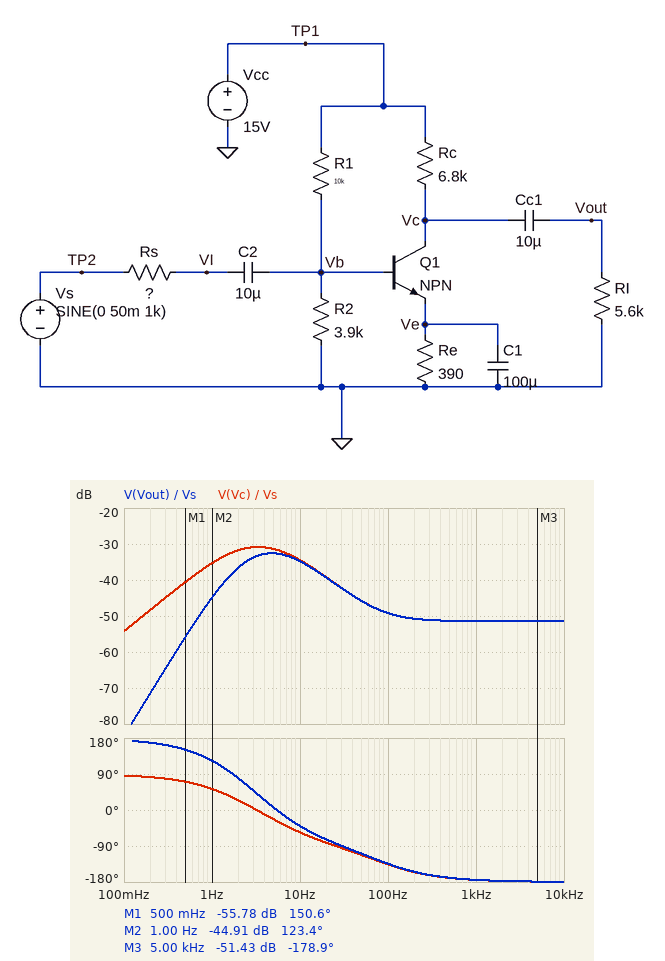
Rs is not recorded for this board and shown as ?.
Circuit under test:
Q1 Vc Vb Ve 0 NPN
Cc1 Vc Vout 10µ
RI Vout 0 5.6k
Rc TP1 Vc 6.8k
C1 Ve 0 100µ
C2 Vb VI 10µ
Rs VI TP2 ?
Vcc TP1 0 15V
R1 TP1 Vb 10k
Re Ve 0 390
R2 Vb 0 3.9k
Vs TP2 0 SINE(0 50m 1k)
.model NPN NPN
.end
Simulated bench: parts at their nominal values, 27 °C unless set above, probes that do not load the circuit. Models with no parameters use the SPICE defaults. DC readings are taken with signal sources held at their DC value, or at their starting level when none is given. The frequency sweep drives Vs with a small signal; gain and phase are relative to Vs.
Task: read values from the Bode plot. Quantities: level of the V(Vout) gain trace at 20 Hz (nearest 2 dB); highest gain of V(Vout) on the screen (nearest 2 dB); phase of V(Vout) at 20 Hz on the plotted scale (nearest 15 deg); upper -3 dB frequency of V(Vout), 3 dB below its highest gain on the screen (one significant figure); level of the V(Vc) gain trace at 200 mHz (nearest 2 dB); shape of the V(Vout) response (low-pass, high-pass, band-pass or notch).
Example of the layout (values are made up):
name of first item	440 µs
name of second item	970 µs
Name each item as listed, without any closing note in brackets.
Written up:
level of the V(Vout) gain trace at 20 Hz	-40 dB
highest gain of V(Vout) on the screen	-32 dB
phase of V(Vout) at 20 Hz on the plotted scale	-75 deg
upper -3 dB frequency of V(Vout), 3 dB below its highest gain on the screen	10 Hz
level of the V(Vc) gain trace at 200 mHz	-48 dB
shape of the V(Vout) response	band-pass
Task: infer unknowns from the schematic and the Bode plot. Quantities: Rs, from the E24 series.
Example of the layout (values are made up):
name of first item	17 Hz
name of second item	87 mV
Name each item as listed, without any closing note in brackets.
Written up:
Rs, from the E24 series	6.8 kΩ
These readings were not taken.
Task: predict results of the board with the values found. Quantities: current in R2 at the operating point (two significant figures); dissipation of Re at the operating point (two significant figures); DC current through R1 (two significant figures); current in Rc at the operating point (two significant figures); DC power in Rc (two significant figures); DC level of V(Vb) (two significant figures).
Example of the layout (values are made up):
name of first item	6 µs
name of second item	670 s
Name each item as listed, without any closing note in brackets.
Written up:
current in R2 at the operating point	490 µA
dissipation of Re at the operating point	3.2 mW
DC current through R1	1.3 mA
current in Rc at the operating point	2.0 mA
DC power in Rc	28 mW
DC level of V(Vb)	1.9 V
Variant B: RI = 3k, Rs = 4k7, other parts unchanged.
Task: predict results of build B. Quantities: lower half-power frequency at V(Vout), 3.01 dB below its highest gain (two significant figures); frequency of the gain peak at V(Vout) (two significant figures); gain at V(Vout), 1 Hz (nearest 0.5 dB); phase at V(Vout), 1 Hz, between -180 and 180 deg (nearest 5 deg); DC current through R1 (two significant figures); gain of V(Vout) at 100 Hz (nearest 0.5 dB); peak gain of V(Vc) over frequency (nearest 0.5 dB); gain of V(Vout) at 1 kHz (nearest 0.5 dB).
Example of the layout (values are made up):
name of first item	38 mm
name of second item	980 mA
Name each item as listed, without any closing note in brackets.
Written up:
lower half-power frequency at V(Vout), 3.01 dB below its highest gain	3.1 Hz
frequency of the gain peak at V(Vout)	6.6 Hz
gain at V(Vout), 1 Hz	-49.5 dB
phase at V(Vout), 1 Hz, between -180 and 180 deg	140 deg
DC current through R1	1.3 mA
gain of V(Vout) at 100 Hz	-46.0 dB
peak gain of V(Vc) over frequency	-29.0 dB
gain of V(Vout) at 1 kHz	-48.0 dB
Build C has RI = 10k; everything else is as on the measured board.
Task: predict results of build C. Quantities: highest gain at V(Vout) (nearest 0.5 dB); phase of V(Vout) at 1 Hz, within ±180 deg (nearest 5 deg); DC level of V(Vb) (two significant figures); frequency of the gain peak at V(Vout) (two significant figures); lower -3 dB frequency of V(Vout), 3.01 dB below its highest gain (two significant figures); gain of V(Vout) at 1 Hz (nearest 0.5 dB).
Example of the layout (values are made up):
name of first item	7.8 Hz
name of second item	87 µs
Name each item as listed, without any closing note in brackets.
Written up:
highest gain at V(Vout)	-31.5 dB
phase of V(Vout) at 1 Hz, within ±180 deg	110 deg
DC level of V(Vb)	1.9 V
frequency of the gain peak at V(Vout)	4.0 Hz
lower -3 dB frequency of V(Vout), 3.01 dB below its highest gain	1.8 Hz
gain of V(Vout) at 1 Hz	-41.0 dB
